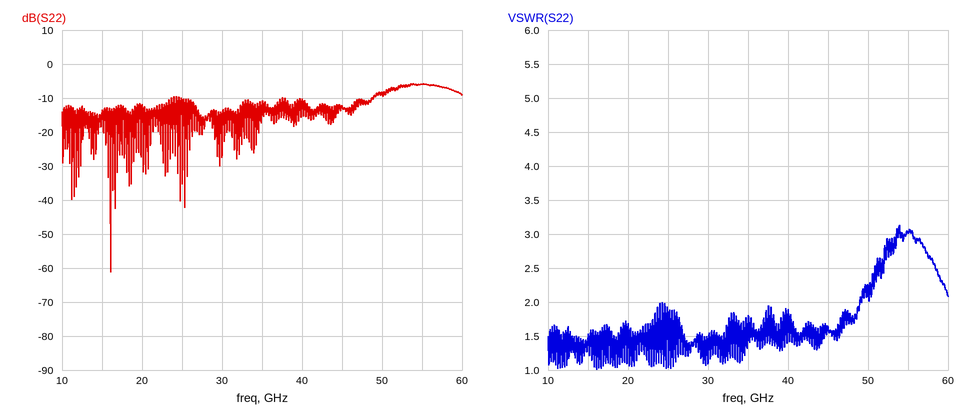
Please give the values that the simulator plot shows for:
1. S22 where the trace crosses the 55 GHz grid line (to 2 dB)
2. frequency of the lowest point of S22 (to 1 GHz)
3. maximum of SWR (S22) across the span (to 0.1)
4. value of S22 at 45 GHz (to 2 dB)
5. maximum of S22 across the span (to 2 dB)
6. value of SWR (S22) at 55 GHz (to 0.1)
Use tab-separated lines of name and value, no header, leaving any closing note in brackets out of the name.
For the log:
S22 where the trace crosses the 55 GHz grid line	-6 dB
frequency of the lowest point of S22	16 GHz
maximum of SWR (S22) across the span	3.1
value of S22 at 45 GHz	-12 dB
maximum of S22 across the span	-6 dB
value of SWR (S22) at 55 GHz	3.0
